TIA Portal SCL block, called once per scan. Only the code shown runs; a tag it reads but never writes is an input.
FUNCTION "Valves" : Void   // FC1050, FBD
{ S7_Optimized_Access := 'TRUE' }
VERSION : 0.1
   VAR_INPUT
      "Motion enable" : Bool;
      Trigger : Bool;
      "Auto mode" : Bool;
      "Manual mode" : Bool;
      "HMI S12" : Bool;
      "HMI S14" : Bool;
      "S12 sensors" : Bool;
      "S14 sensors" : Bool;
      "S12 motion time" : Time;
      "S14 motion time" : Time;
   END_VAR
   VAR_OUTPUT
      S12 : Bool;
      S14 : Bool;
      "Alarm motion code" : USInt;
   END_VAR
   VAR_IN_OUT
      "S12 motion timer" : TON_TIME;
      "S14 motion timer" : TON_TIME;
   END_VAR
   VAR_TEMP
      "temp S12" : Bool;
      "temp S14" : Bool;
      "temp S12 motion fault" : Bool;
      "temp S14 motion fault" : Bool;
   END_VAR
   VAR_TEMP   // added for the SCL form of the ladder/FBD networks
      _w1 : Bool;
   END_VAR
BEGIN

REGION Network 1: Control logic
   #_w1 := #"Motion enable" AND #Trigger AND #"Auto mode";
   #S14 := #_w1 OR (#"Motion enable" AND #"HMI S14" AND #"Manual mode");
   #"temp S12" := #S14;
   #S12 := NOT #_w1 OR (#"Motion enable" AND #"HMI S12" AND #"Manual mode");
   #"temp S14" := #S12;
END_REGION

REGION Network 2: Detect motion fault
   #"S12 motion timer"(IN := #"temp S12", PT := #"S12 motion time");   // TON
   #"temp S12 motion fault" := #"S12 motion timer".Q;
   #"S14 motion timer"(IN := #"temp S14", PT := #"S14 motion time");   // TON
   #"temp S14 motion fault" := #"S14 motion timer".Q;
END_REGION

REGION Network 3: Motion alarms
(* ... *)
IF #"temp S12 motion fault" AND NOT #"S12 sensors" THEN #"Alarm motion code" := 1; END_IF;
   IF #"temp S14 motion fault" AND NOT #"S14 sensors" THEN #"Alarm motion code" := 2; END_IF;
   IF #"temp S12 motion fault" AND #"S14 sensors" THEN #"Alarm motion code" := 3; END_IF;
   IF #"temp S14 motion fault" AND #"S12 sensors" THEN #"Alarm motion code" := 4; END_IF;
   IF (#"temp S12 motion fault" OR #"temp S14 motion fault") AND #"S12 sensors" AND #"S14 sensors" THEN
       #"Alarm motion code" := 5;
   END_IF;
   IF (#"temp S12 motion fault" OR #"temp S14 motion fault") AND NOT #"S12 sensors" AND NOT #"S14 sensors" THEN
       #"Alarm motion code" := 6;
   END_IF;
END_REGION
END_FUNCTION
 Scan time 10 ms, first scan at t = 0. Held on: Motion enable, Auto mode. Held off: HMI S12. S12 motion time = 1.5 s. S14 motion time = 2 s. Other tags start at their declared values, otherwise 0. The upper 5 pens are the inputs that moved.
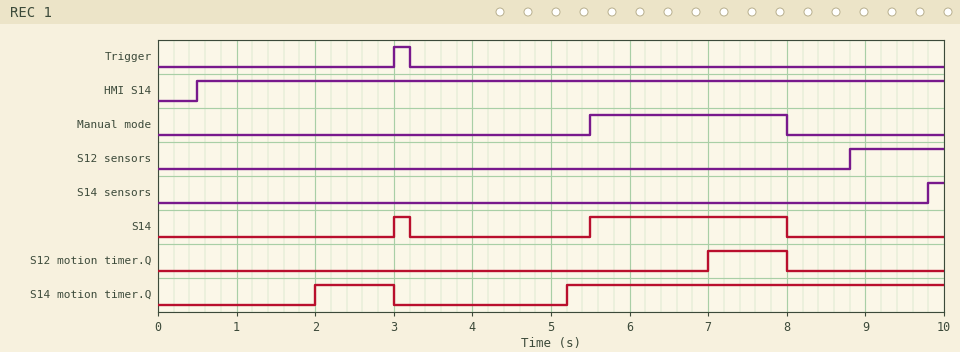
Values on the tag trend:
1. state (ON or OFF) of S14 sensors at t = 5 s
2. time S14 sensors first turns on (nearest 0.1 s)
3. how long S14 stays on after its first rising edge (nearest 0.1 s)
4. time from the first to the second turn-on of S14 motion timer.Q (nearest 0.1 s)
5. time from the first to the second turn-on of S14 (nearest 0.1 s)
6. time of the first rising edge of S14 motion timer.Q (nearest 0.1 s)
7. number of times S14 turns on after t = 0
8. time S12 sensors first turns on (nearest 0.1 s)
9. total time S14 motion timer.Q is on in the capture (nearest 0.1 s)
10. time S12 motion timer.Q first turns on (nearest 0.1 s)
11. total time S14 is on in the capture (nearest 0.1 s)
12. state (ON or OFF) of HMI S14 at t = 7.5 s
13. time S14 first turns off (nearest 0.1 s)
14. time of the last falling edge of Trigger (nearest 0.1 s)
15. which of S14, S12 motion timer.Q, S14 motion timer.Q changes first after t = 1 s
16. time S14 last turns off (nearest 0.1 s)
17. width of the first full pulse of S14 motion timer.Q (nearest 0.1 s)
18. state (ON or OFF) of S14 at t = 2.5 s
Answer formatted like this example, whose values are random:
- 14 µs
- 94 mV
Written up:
- OFF
- 9.8 s
- 0.2 s
- 3.2 s
- 2.5 s
- 2.0 s
- 2
- 8.8 s
- 5.8 s
- 7.0 s
- 2.7 s
- ON
- 3.2 s
- 3.2 s
- S14 motion timer.Q
- 8.0 s
- 1.0 s
- OFF
